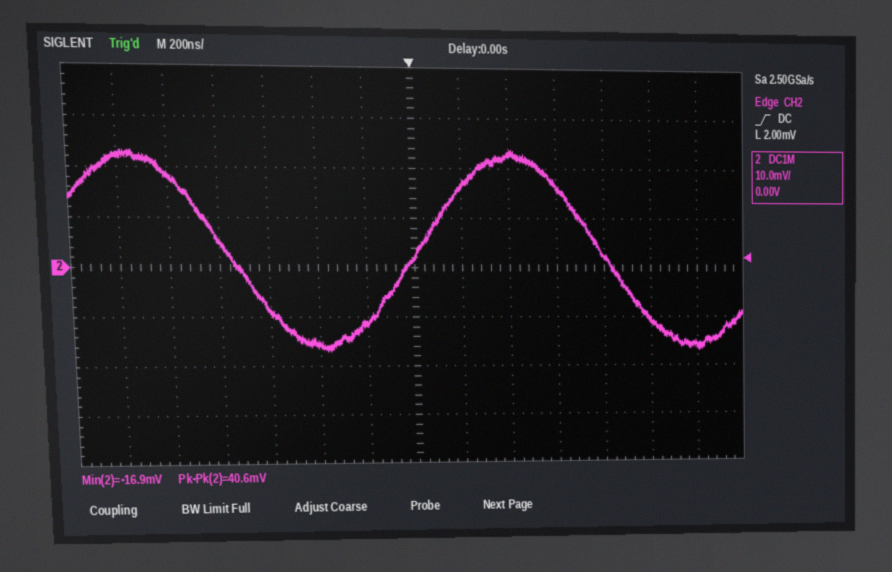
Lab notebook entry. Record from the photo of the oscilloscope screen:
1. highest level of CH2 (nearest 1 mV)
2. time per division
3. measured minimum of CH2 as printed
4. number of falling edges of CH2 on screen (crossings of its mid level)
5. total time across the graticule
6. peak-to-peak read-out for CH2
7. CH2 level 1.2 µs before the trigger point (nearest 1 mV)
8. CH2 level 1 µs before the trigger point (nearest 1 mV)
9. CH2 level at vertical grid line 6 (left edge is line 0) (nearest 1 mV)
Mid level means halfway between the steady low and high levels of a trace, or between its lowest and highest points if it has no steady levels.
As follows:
24 mV
200 ns
-16.9 mV
2
2.8 µs
40.6 mV
22 mV
18 mV
-11 mV
